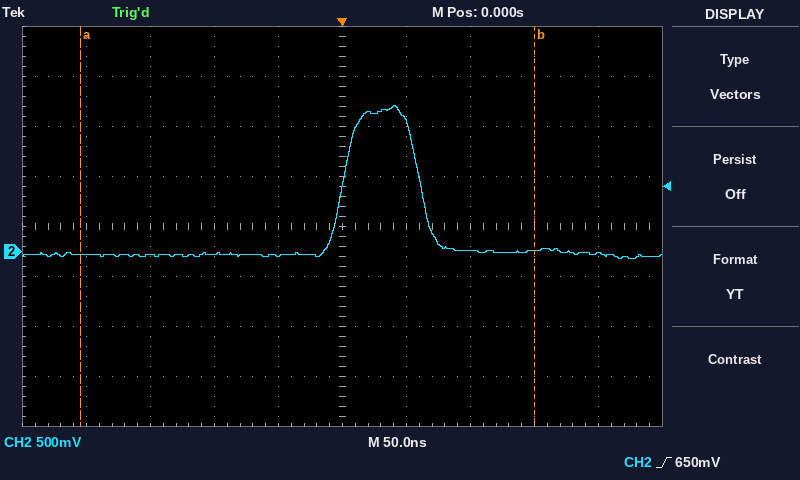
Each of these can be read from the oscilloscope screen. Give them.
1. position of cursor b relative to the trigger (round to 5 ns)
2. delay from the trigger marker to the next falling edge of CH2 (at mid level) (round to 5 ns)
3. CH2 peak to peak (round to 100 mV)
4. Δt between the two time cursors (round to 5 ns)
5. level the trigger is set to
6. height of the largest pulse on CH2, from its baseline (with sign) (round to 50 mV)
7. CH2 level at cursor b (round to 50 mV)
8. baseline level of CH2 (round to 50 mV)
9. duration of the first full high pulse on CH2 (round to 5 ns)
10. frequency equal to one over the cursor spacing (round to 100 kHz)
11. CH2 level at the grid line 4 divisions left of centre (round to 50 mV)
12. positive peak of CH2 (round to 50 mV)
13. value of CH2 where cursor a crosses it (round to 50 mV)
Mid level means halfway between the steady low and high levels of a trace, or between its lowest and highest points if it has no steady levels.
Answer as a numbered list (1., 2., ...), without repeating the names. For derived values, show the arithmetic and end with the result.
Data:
1. +150 ns
2. 60 ns
3. 1.50 V
4. 355 ns
5. 650 mV
6. 1.45 V − (-50 mV) = +1.50 V
7. 0 mV
8. -50 mV
9. 60 ns
10. 1 / 355 ns ≈ 2.8 MHz
11. -50 mV
12. 1.45 V
13. -50 mV
